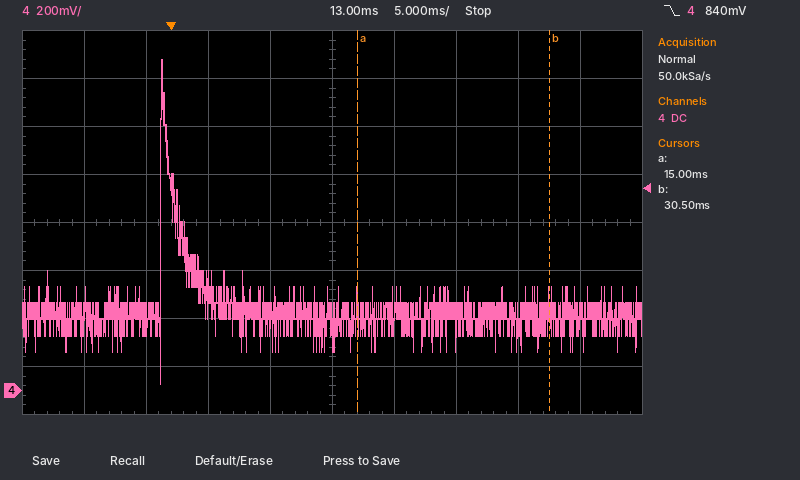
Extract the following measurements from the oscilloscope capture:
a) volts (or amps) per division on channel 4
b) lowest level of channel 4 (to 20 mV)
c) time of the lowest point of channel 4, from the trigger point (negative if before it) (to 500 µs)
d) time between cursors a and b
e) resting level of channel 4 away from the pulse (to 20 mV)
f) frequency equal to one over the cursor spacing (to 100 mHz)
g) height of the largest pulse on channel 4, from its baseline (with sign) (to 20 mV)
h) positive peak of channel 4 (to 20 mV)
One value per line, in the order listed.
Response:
200 mV
20 mV
-1.0 ms
15.5 ms
300 mV
64.5 Hz
+1.08 V
1.38 V
